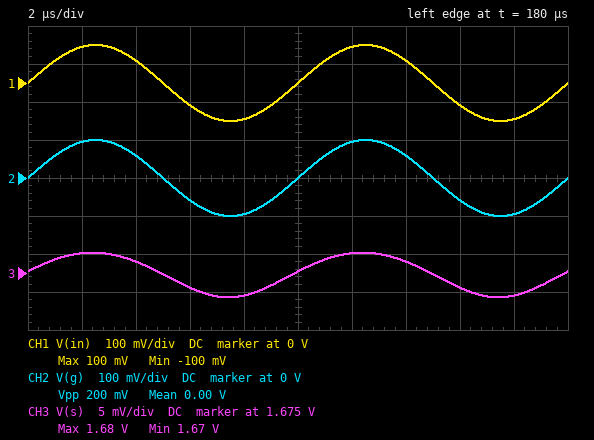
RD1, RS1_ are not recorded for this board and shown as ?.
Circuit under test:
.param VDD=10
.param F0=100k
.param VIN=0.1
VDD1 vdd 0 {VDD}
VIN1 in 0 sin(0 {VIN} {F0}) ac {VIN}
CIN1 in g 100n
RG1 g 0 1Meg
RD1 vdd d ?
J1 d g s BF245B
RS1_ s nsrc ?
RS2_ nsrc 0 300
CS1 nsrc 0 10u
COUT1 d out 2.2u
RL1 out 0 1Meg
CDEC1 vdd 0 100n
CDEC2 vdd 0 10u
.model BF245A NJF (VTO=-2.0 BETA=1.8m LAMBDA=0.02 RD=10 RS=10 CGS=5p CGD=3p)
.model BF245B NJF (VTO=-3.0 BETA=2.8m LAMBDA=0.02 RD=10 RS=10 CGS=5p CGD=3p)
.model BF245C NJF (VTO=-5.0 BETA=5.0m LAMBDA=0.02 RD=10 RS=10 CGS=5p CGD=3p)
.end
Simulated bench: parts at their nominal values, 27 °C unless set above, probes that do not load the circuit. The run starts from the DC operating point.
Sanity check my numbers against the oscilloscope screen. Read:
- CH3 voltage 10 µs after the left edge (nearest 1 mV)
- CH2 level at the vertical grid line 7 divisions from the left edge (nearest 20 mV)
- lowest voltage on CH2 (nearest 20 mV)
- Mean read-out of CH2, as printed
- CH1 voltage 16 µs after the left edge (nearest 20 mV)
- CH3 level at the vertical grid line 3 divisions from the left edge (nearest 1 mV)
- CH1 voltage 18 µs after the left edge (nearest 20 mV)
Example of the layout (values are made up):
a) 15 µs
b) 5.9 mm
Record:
a) 1.675 V
b) 60 mV
c) -100 mV
d) 0.00 V
e) -60 mV
f) 1.673 V
g) -100 mV
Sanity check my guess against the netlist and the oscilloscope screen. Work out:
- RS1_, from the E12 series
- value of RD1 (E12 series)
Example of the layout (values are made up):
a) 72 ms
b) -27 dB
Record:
a) 680 Ω
b) 4.7 kΩ
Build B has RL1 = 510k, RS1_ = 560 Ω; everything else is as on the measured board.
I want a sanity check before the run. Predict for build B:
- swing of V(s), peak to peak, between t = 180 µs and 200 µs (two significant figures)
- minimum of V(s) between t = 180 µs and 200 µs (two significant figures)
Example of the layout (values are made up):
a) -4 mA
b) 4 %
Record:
a) 3.8 mV
b) 1.5 V
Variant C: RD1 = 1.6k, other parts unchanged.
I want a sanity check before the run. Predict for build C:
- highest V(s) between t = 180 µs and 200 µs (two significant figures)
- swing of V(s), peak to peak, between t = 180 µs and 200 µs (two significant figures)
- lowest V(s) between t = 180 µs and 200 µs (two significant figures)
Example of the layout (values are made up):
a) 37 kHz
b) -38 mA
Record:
a) 2.2 V
b) 150 mV
c) 2.1 V
